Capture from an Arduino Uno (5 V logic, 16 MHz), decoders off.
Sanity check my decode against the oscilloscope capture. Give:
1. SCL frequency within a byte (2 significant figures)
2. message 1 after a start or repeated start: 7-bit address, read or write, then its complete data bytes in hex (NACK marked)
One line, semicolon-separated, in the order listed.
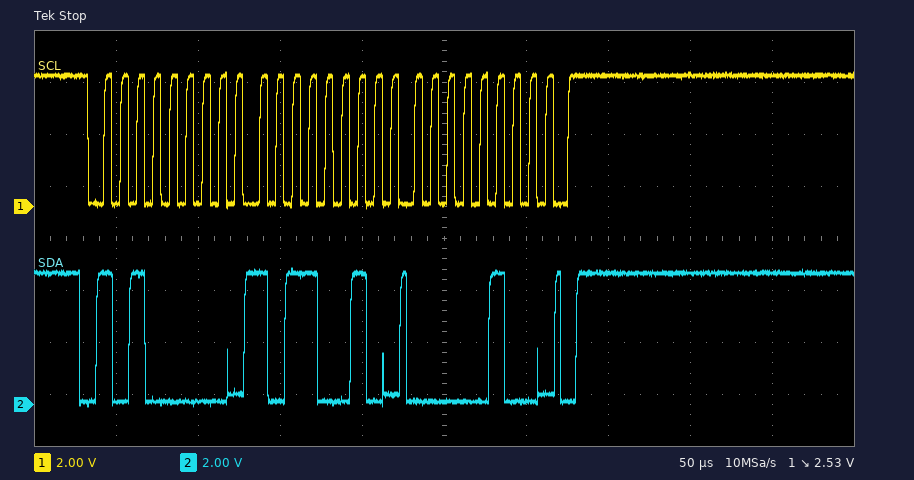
100 kHz; 0x50 write: B2 04
